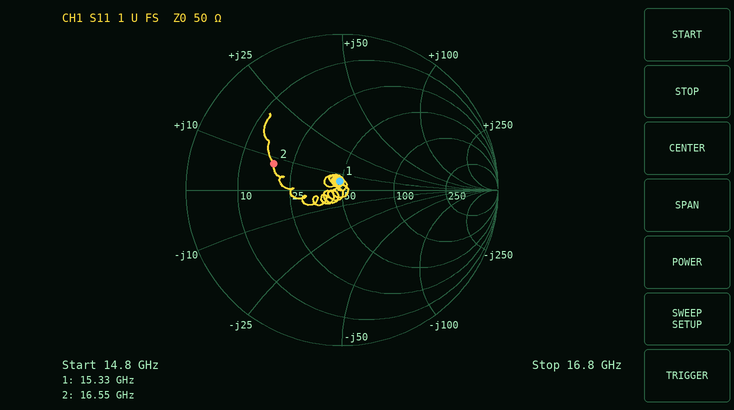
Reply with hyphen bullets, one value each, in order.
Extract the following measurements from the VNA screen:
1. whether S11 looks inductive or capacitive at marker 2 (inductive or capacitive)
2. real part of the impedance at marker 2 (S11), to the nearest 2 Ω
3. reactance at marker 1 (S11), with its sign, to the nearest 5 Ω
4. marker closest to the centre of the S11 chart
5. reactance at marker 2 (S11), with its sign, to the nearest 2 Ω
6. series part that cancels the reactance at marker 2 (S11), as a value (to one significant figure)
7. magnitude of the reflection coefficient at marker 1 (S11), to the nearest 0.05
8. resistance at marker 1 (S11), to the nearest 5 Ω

- inductive
- 18 Ω
- +5 Ω
- marker 1
- +8 Ω
- 1 pF
- 0.05
- 50 Ω
